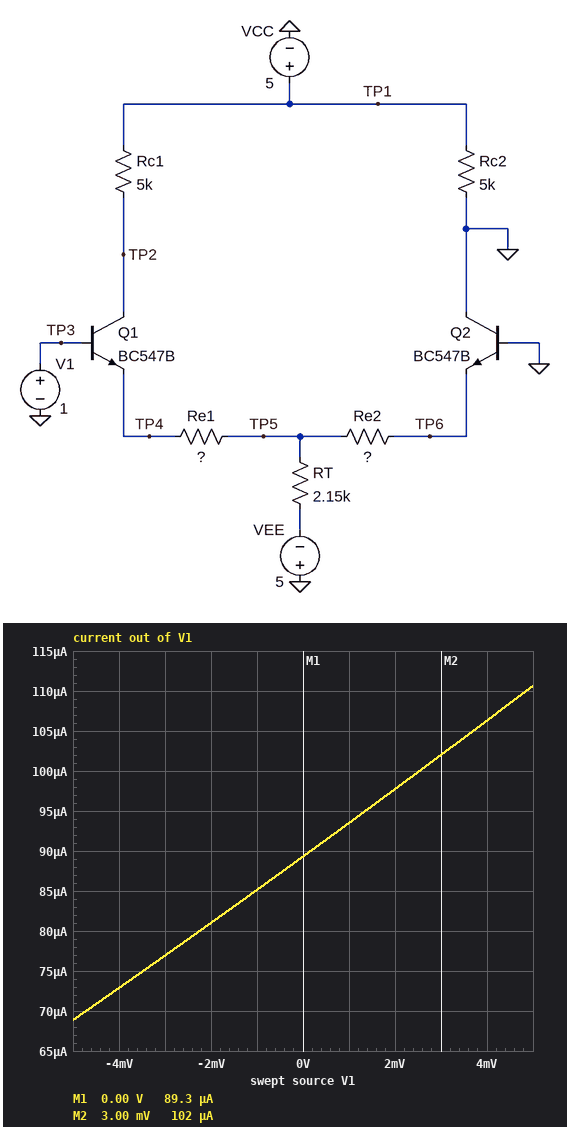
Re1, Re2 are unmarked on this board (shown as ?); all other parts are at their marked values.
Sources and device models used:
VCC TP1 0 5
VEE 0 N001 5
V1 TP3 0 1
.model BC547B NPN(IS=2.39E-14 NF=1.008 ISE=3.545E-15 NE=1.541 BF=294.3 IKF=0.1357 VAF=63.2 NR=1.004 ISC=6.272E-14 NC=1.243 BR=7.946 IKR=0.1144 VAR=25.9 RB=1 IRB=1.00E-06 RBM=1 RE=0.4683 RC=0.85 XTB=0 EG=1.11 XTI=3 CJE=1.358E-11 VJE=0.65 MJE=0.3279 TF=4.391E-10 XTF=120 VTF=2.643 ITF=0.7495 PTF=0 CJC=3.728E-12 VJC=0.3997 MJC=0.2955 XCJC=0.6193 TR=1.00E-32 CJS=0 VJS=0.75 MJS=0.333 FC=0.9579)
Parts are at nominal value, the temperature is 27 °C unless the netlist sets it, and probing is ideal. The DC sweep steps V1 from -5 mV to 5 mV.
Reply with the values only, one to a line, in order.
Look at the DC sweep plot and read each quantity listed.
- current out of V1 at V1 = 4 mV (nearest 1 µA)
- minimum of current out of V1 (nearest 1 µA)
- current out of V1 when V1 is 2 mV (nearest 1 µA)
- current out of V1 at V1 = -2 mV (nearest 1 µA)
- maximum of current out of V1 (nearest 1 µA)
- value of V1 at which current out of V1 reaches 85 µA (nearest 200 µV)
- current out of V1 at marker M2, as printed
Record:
106 µA
69 µA
98 µA
81 µA
111 µA
-1.0 mV
102 µA
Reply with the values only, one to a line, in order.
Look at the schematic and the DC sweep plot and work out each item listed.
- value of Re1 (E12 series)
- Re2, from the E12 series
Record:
27 Ω
68 Ω
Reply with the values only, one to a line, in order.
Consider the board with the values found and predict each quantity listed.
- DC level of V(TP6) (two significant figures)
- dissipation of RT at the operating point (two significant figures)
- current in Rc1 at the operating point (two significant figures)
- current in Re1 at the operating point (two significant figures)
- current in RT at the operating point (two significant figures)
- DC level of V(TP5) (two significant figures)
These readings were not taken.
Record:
230 mV
13 mW
940 µA
2.4 mA
2.4 mA
230 mV
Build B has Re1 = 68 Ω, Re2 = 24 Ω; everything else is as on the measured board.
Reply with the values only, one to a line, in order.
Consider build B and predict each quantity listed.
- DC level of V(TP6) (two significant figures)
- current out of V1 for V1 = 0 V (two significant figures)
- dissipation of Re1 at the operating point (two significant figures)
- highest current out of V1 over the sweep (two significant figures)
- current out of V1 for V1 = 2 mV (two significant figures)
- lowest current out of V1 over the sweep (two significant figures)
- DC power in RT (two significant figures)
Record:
130 mV
2.4 µA
390 µW
2.6 µA
2.5 µA
2.3 µA
12 mW
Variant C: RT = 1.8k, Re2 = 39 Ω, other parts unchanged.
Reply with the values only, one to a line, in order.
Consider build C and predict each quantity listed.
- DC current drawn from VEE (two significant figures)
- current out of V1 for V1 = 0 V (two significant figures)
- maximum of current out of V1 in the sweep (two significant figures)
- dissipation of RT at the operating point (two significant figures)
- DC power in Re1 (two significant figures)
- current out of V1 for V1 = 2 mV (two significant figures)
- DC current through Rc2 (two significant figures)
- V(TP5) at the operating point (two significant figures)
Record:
2.9 mA
100 µA
130 µA
15 mW
230 µW
110 µA
1.0 mA
210 mV
